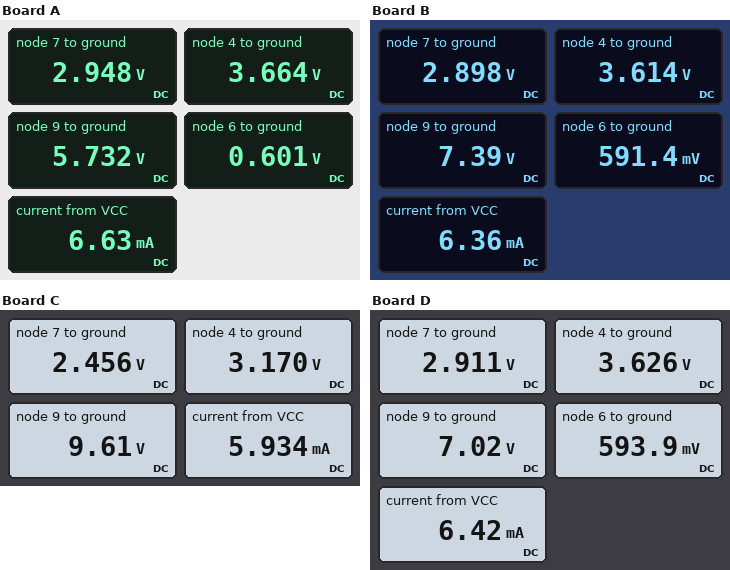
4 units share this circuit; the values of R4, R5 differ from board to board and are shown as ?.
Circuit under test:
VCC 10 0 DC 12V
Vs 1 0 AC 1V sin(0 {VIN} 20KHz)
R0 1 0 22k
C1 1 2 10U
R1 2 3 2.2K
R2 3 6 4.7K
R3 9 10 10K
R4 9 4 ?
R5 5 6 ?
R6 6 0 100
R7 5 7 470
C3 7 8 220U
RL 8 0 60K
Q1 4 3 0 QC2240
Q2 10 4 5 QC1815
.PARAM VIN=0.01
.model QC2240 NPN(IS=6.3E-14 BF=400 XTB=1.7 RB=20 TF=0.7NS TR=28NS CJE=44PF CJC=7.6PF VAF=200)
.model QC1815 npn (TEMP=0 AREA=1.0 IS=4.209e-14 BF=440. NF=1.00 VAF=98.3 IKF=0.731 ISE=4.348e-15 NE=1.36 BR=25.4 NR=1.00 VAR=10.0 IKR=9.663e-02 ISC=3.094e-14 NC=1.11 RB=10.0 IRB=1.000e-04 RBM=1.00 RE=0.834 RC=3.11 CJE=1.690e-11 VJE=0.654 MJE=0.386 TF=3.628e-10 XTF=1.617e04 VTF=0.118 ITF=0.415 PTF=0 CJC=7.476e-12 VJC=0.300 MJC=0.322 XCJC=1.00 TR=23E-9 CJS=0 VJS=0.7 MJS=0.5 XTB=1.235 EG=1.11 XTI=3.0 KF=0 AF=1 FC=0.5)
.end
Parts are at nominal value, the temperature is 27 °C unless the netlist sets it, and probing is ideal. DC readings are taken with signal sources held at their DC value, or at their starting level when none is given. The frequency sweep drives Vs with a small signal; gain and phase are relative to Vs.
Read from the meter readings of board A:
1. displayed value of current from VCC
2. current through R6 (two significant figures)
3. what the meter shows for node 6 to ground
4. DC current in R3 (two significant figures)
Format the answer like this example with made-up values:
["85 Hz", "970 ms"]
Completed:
["6.63 mA", "6.0 mA", "0.601 V", "630 µA"]
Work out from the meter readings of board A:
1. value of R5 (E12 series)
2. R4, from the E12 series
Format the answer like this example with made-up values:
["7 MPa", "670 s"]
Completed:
["390 Ω", "3.3 kΩ"]
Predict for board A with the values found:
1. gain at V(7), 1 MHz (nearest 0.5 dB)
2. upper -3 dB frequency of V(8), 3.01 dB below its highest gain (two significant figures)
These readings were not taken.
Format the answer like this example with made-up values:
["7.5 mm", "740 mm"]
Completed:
["18.5 dB", "1.5 MHz"]
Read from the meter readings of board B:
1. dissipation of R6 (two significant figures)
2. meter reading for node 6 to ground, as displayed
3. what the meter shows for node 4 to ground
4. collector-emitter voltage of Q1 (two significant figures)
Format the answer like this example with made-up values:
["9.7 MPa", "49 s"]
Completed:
["3.5 mW", "591.4 mV", "3.614 V", "3.6 V"]
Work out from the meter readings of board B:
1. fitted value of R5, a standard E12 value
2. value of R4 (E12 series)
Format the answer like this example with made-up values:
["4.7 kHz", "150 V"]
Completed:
["390 Ω", "8.2 kΩ"]
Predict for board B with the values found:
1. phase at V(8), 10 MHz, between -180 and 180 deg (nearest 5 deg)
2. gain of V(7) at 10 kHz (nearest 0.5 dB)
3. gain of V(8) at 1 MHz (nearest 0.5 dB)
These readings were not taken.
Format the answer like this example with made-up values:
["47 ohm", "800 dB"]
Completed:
["70 deg", "20.0 dB", "18.5 dB"]
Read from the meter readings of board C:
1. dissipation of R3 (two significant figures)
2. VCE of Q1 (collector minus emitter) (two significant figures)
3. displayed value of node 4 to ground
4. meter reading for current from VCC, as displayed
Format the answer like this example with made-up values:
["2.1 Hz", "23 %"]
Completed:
["570 µW", "3.2 V", "3.170 V", "5.934 mA"]
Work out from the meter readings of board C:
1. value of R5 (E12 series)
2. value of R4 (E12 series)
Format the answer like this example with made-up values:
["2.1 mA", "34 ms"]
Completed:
["330 Ω", "27 kΩ"]
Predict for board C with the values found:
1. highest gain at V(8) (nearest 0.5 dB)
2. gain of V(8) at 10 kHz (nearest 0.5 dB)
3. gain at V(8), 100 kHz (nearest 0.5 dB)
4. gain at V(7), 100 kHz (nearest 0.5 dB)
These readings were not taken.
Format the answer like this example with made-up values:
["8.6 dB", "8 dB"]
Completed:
["19.0 dB", "19.0 dB", "19.0 dB", "19.0 dB"]
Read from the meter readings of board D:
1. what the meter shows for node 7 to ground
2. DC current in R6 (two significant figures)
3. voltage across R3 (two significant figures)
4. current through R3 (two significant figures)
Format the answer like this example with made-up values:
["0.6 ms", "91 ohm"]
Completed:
["2.911 V", "5.9 mA", "5.0 V", "500 µA"]
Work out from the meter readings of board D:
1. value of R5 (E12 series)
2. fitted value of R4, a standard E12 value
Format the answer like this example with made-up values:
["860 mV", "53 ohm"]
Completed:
["390 Ω", "6.8 kΩ"]
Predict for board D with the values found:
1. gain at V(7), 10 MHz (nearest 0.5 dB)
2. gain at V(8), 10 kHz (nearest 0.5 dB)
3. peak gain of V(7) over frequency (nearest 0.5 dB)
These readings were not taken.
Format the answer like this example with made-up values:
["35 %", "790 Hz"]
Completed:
["2.5 dB", "20.0 dB", "20.0 dB"]
